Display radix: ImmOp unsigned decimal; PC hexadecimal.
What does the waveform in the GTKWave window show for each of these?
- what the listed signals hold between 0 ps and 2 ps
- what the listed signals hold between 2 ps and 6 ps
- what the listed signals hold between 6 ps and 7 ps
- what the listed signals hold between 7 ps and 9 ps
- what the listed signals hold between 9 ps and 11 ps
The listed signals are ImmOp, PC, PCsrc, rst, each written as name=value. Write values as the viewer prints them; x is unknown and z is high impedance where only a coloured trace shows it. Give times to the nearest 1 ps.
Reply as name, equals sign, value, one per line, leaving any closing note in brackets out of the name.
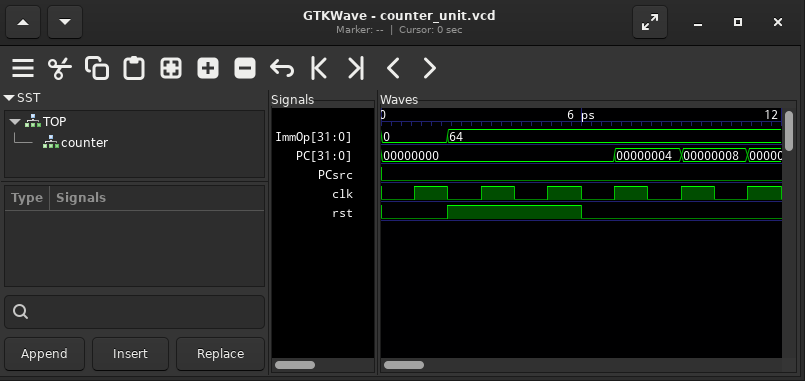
what the listed signals hold between 0 ps and 2 ps = ImmOp=0, PC=00000000, PCsrc=0, rst=0
what the listed signals hold between 2 ps and 6 ps = ImmOp=64, PC=00000000, PCsrc=0, rst=1
what the listed signals hold between 6 ps and 7 ps = ImmOp=64, PC=00000000, PCsrc=0, rst=0
what the listed signals hold between 7 ps and 9 ps = ImmOp=64, PC=00000004, PCsrc=0, rst=0
what the listed signals hold between 9 ps and 11 ps = ImmOp=64, PC=00000008, PCsrc=0, rst=0
